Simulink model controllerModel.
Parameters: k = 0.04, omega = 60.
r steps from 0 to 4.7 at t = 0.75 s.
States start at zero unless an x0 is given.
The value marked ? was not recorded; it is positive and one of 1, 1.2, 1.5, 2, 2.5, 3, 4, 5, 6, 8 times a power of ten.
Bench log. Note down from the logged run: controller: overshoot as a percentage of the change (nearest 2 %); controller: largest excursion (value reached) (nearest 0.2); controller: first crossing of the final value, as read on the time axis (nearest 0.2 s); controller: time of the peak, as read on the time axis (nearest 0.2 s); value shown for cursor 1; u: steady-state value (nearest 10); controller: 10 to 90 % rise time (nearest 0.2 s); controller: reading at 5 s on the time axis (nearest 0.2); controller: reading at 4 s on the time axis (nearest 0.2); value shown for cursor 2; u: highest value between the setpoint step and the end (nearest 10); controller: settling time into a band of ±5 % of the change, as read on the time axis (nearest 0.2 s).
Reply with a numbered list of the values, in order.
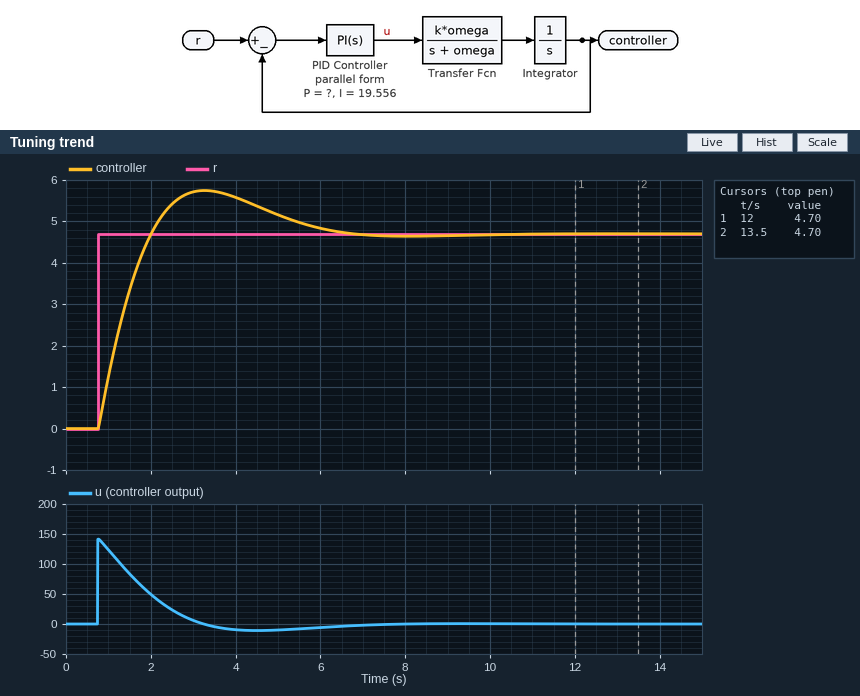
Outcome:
1. 22 %
2. 5.8
3. 2.0 s
4. 3.2 s
5. 4.70
6. 0
7. 1.0 s
8. 5.2
9. 5.6
10. 4.70
11. 140
12. 5.6 s
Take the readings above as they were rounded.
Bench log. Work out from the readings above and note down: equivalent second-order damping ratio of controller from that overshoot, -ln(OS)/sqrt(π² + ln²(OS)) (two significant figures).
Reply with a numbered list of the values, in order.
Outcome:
1. 0.43
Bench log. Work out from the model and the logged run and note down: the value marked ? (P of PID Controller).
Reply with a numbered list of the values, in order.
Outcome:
1. 30
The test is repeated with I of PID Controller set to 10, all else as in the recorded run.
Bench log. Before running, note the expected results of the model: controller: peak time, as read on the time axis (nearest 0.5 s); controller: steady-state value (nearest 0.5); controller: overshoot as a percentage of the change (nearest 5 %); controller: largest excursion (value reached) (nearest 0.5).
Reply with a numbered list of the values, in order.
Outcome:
1. 4.0 s
2. 4.5
3. 15 %
4. 5.5
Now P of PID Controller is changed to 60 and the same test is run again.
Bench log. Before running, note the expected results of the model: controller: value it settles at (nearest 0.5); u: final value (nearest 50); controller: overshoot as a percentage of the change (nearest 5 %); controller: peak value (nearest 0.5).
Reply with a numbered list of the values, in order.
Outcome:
1. 4.5
2. 0
3. 10 %
4. 5.0
